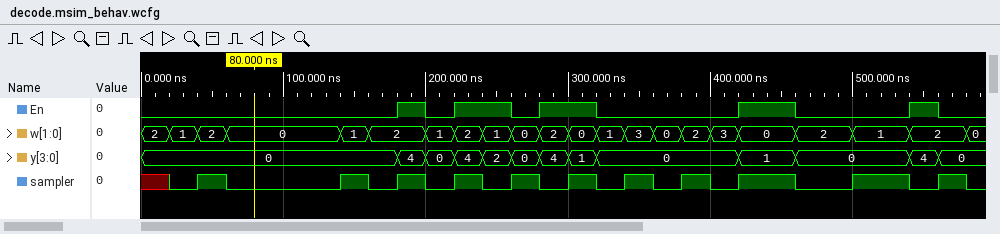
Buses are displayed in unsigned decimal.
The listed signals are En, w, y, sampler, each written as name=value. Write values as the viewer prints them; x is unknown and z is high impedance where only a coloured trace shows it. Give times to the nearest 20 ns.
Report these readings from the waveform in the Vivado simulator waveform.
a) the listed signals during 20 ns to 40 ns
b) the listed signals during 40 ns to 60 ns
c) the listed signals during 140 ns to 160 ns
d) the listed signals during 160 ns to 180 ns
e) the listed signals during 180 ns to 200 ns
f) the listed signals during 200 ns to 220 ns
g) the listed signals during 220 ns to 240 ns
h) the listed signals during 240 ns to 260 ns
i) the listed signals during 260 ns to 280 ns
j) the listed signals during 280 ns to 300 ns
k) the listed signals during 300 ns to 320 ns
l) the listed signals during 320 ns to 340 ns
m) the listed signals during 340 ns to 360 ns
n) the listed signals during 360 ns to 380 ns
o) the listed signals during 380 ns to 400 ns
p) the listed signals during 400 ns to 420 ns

En=0, w=1, y=0, sampler=0
En=0, w=2, y=0, sampler=1
En=0, w=1, y=0, sampler=1
En=0, w=2, y=0, sampler=0
En=1, w=2, y=4, sampler=1
En=0, w=1, y=0, sampler=0
En=1, w=2, y=4, sampler=1
En=1, w=1, y=2, sampler=0
En=0, w=0, y=0, sampler=1
En=1, w=2, y=4, sampler=0
En=1, w=0, y=1, sampler=1
En=0, w=1, y=0, sampler=0
En=0, w=3, y=0, sampler=1
En=0, w=0, y=0, sampler=0
En=0, w=2, y=0, sampler=1
En=0, w=3, y=0, sampler=0
